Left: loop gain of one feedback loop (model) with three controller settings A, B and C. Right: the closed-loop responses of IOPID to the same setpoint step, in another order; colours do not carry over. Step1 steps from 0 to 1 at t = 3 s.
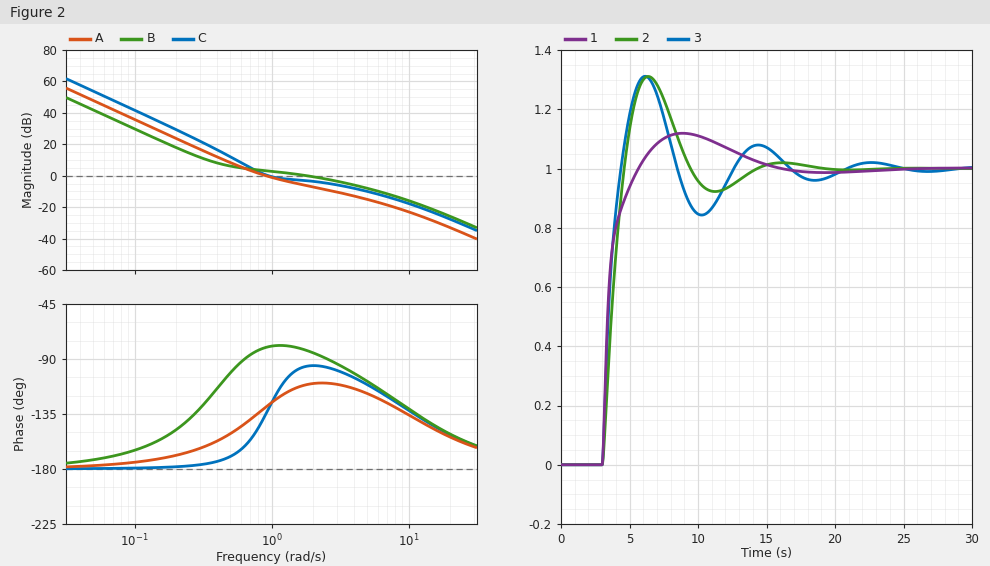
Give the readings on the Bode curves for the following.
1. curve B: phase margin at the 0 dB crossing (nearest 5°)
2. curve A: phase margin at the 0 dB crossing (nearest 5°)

95°
50°
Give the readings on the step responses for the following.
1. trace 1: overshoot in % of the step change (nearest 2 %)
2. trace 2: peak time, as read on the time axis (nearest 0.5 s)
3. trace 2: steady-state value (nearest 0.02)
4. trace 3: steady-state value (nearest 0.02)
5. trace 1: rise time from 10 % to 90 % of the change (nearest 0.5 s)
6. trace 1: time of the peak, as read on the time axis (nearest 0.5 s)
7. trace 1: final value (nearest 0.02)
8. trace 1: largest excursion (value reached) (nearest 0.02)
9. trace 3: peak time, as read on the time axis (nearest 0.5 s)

12 %
6.5 s
1.00
1.00
1.5 s
9.0 s
1.00
1.12
6.0 s
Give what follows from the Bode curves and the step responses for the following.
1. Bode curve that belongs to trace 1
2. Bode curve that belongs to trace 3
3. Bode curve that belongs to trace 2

B
C
A
